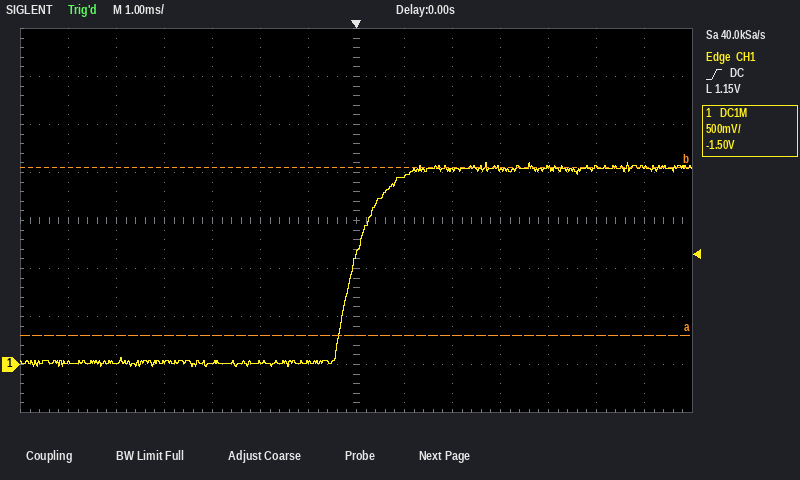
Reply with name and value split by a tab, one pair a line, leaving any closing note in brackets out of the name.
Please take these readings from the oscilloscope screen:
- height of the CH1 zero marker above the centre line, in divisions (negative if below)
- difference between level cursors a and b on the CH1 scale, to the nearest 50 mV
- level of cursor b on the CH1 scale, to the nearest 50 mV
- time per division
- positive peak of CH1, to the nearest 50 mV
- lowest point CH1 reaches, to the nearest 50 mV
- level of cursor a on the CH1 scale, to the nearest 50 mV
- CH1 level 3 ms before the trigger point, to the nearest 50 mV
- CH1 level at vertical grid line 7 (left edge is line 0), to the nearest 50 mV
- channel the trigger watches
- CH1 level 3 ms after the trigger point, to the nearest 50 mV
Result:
height of the CH1 zero marker above the centre line, in divisions	-3.0 div
difference between level cursors a and b on the CH1 scale, to the nearest 50 mV	1.75 V
level of cursor b on the CH1 scale, to the nearest 50 mV	2.05 V
time per division	1 ms
positive peak of CH1, to the nearest 50 mV	2.10 V
lowest point CH1 reaches, to the nearest 50 mV	0 mV
level of cursor a on the CH1 scale, to the nearest 50 mV	300 mV
CH1 level 3 ms before the trigger point, to the nearest 50 mV	0 mV
CH1 level at vertical grid line 7 (left edge is line 0), to the nearest 50 mV	1.15 V
channel the trigger watches	CH1
CH1 level 3 ms after the trigger point, to the nearest 50 mV	2.05 V
